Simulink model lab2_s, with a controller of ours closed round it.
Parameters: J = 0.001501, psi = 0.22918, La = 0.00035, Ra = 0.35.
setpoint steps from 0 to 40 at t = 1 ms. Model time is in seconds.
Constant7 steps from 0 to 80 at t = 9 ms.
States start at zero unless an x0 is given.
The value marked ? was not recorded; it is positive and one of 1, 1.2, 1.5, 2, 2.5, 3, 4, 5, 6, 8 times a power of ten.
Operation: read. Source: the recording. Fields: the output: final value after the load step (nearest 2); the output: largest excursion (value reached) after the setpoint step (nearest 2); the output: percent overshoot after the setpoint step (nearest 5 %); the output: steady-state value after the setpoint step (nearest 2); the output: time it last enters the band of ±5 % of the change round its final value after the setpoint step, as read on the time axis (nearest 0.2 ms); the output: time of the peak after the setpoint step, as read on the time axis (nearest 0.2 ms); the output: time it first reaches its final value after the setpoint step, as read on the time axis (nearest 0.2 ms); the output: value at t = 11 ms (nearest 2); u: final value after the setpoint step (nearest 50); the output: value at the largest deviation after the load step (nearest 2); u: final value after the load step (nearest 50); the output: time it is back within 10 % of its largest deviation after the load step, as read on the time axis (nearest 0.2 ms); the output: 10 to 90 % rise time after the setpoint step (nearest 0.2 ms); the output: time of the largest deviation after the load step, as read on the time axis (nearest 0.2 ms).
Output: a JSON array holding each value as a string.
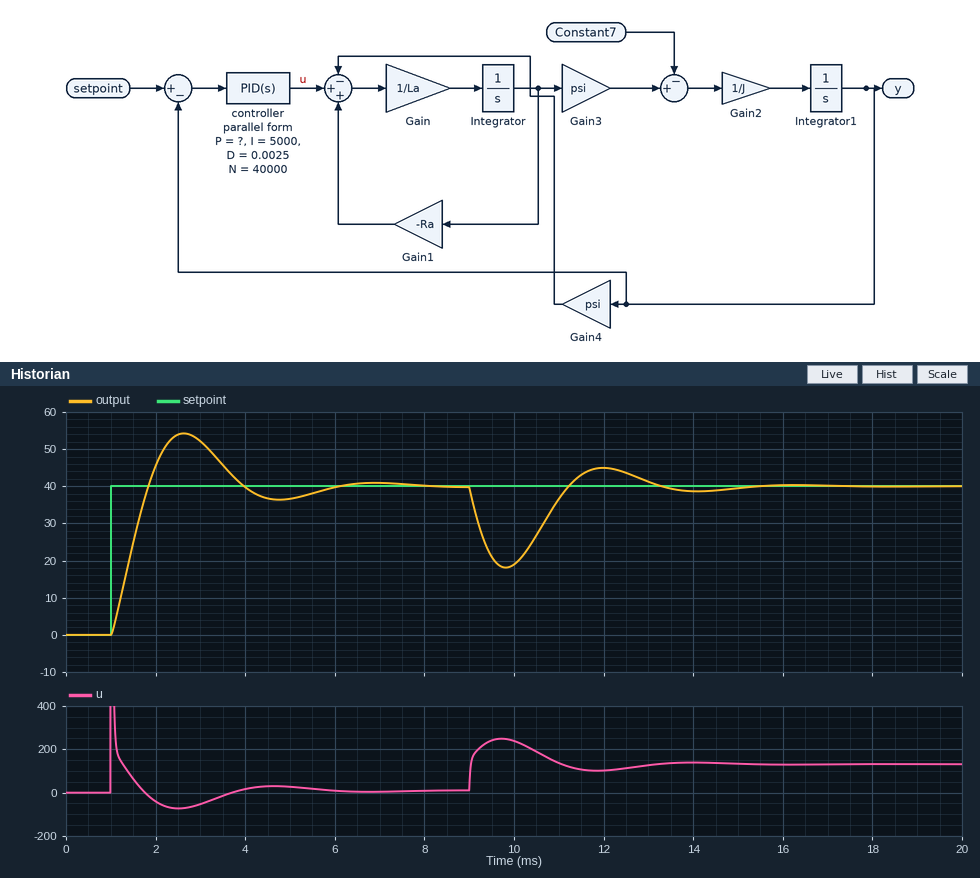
["40", "54", "35 %", "40", "5.4 ms", "2.6 ms", "1.8 ms", "36", "0", "18", "150", "12.8 ms", "0.6 ms", "9.8 ms"]
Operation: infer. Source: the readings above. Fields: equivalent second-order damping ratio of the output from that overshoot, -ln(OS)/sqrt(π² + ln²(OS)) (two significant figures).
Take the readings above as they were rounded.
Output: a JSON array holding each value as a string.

["0.32"]
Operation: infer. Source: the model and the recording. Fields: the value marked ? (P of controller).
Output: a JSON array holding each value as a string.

["8"]
